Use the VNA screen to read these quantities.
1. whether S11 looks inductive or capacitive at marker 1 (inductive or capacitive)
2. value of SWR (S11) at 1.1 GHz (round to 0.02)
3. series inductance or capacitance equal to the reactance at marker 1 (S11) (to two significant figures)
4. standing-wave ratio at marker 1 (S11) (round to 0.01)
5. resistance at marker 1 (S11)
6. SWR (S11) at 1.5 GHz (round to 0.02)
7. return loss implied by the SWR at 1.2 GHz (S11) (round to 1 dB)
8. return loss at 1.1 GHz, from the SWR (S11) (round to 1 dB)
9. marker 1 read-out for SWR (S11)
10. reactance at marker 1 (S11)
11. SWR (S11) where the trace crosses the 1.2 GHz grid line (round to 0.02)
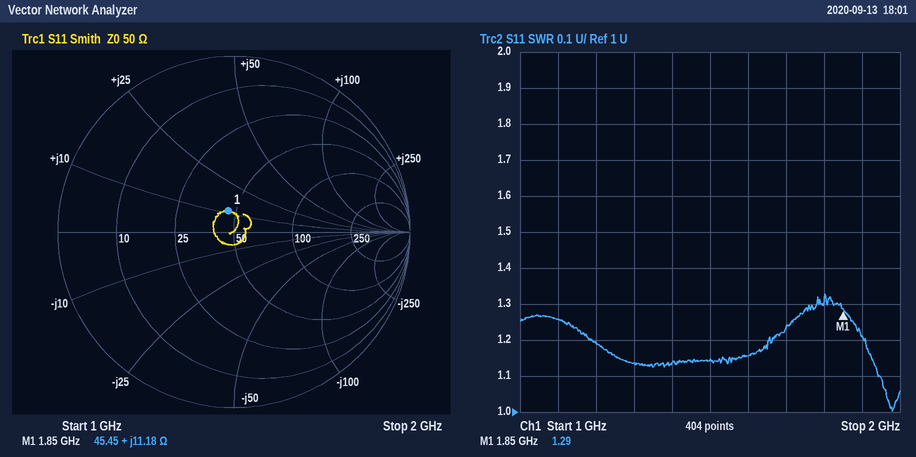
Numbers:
inductive
1.26
960 pH
1.29
45.45 Ω
1.14
21 dB
19 dB
1.29
+11.18 Ω
1.20
